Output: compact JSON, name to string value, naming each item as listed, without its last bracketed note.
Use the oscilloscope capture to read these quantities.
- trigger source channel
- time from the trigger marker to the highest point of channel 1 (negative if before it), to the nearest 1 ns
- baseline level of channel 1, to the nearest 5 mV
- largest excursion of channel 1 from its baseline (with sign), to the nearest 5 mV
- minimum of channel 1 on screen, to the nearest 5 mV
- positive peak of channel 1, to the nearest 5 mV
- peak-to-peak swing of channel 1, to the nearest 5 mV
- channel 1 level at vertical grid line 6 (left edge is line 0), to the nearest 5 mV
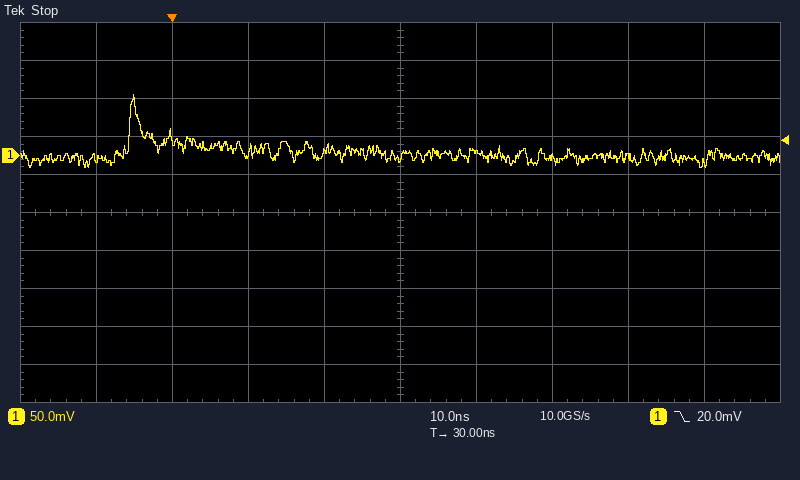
{"trigger source channel": "channel 1", "time from the trigger marker to the highest point of channel 1 (negative if before it), to the nearest 1 ns": "-5 ns", "baseline level of channel 1, to the nearest 5 mV": "0 mV", "largest excursion of channel 1 from its baseline (with sign), to the nearest 5 mV": "+80 mV", "minimum of channel 1 on screen, to the nearest 5 mV": "-15 mV", "positive peak of channel 1, to the nearest 5 mV": "80 mV", "peak-to-peak swing of channel 1, to the nearest 5 mV": "95 mV", "channel 1 level at vertical grid line 6 (left edge is line 0), to the nearest 5 mV": "5 mV"}
